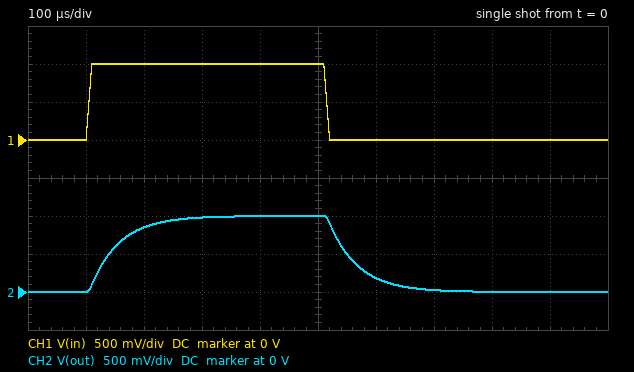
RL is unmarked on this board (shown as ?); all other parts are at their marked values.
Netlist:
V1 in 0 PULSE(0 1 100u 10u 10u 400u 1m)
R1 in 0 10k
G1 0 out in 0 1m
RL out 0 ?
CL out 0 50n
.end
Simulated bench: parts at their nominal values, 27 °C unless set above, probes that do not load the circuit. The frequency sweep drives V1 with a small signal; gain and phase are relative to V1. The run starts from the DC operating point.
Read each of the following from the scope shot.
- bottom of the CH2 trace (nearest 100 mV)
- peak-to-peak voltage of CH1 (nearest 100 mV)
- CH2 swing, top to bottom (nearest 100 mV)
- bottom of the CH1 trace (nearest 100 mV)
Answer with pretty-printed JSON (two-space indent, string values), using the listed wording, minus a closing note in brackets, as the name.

{
  "bottom of the CH2 trace": "0 V",
  "peak-to-peak voltage of CH1": "1.0 V",
  "CH2 swing, top to bottom": "1.0 V",
  "bottom of the CH1 trace": "0 V"
}
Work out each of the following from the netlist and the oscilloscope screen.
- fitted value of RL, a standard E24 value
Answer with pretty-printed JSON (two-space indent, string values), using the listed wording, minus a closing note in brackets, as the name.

{
  "fitted value of RL, a standard E24 value": "1 kΩ"
}
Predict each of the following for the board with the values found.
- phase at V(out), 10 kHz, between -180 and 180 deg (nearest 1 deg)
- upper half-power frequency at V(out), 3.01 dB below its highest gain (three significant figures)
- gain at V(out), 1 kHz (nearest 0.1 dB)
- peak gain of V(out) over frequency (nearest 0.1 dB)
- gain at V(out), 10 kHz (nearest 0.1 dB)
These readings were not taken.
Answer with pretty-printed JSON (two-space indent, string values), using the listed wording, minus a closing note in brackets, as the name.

{
  "phase at V(out), 10 kHz, between -180 and 180 deg": "-72 deg",
  "upper half-power frequency at V(out), 3.01 dB below its highest gain": "3.18 kHz",
  "gain at V(out), 1 kHz": "-0.4 dB",
  "peak gain of V(out) over frequency": "0 dB",
  "gain at V(out), 10 kHz": "-10.4 dB"
}
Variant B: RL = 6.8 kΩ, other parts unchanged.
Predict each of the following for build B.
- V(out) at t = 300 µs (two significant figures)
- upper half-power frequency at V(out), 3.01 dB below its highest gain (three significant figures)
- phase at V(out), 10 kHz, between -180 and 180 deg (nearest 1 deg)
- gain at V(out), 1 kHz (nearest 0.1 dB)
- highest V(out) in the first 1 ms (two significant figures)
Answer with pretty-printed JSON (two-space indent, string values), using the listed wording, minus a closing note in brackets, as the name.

{
  "V(out) at t = 300 µs": "3.0 V",
  "upper half-power frequency at V(out), 3.01 dB below its highest gain": "468 Hz",
  "phase at V(out), 10 kHz, between -180 and 180 deg": "-87 deg",
  "gain at V(out), 1 kHz": "9.2 dB",
  "highest V(out) in the first 1 ms": "4.7 V"
}
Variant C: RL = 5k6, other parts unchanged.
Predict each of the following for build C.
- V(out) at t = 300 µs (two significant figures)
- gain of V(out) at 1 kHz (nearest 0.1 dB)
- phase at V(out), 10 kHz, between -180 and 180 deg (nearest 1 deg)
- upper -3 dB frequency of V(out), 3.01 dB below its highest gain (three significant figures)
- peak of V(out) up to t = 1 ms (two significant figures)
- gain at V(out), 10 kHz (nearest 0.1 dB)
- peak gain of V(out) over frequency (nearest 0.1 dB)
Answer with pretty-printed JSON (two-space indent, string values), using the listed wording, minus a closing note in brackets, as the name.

{
  "V(out) at t = 300 µs": "2.8 V",
  "gain of V(out) at 1 kHz": "8.8 dB",
  "phase at V(out), 10 kHz, between -180 and 180 deg": "-87 deg",
  "upper -3 dB frequency of V(out), 3.01 dB below its highest gain": "568 Hz",
  "peak of V(out) up to t = 1 ms": "4.3 V",
  "gain at V(out), 10 kHz": "-10.0 dB",
  "peak gain of V(out) over frequency": "15.0 dB"
}
